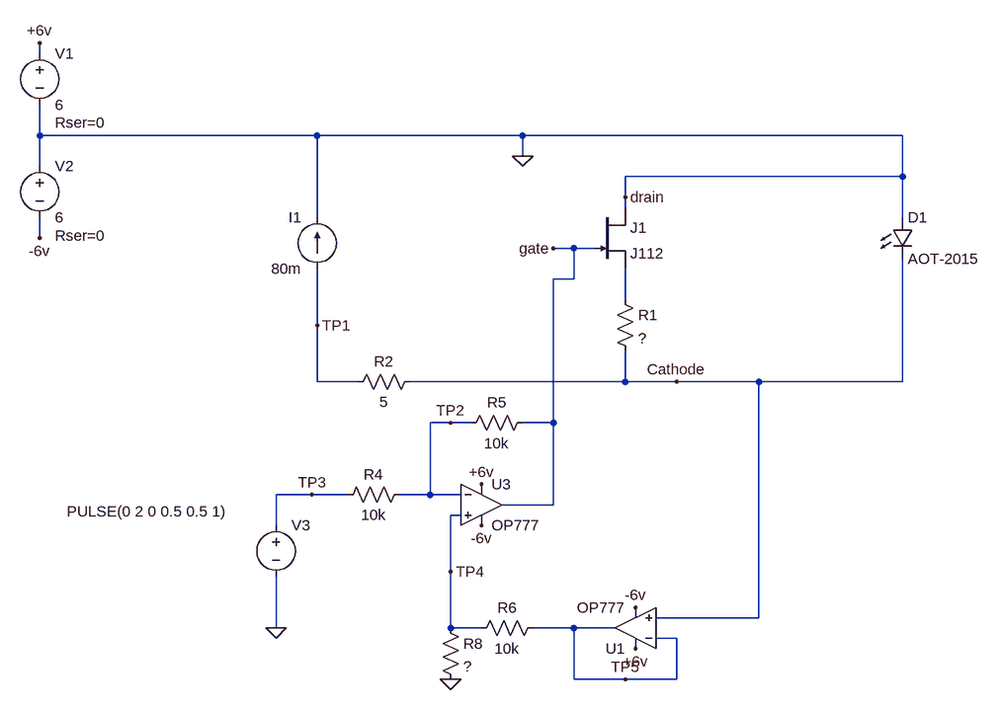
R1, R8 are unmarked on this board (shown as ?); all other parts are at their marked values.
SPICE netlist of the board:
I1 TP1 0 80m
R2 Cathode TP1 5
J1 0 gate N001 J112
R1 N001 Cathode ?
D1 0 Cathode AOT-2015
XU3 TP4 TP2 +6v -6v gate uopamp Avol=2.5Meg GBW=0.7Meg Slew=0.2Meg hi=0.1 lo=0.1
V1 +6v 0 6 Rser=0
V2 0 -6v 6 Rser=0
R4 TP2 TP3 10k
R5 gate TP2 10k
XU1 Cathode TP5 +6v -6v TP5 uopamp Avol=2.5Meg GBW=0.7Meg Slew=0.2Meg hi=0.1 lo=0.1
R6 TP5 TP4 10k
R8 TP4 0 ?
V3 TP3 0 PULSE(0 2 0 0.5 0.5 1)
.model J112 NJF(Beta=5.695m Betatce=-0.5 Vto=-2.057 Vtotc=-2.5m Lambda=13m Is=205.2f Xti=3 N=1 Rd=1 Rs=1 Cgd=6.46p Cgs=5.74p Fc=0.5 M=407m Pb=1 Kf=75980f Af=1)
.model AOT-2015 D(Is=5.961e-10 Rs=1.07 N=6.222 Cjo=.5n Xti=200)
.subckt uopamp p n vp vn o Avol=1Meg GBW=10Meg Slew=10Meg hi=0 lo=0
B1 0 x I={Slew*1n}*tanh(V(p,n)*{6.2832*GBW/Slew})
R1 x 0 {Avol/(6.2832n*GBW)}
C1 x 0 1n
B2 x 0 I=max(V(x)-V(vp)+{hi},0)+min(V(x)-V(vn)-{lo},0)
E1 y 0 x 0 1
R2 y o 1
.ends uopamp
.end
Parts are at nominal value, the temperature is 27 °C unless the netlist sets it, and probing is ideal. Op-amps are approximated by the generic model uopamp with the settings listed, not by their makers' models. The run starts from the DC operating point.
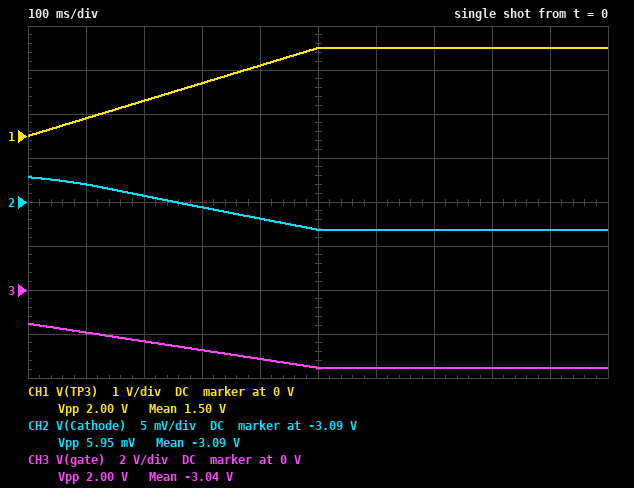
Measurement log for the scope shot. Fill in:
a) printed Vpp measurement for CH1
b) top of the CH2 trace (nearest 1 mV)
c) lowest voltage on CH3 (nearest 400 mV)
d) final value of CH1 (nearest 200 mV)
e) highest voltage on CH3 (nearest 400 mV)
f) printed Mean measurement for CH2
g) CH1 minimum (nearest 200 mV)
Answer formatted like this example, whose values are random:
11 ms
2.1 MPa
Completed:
2.00 V
-3.087 V
-3.6 V
2.0 V
-1.6 V
-3.09 V
0 V
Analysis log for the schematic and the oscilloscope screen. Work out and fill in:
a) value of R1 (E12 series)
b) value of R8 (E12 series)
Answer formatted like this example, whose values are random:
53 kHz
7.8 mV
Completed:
820 Ω
3.3 kΩ
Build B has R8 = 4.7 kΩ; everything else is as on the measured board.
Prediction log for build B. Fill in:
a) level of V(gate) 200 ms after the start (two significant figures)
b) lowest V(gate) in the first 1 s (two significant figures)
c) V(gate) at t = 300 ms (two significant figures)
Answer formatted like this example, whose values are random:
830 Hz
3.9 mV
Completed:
-2.8 V
-4.0 V
-3.2 V
